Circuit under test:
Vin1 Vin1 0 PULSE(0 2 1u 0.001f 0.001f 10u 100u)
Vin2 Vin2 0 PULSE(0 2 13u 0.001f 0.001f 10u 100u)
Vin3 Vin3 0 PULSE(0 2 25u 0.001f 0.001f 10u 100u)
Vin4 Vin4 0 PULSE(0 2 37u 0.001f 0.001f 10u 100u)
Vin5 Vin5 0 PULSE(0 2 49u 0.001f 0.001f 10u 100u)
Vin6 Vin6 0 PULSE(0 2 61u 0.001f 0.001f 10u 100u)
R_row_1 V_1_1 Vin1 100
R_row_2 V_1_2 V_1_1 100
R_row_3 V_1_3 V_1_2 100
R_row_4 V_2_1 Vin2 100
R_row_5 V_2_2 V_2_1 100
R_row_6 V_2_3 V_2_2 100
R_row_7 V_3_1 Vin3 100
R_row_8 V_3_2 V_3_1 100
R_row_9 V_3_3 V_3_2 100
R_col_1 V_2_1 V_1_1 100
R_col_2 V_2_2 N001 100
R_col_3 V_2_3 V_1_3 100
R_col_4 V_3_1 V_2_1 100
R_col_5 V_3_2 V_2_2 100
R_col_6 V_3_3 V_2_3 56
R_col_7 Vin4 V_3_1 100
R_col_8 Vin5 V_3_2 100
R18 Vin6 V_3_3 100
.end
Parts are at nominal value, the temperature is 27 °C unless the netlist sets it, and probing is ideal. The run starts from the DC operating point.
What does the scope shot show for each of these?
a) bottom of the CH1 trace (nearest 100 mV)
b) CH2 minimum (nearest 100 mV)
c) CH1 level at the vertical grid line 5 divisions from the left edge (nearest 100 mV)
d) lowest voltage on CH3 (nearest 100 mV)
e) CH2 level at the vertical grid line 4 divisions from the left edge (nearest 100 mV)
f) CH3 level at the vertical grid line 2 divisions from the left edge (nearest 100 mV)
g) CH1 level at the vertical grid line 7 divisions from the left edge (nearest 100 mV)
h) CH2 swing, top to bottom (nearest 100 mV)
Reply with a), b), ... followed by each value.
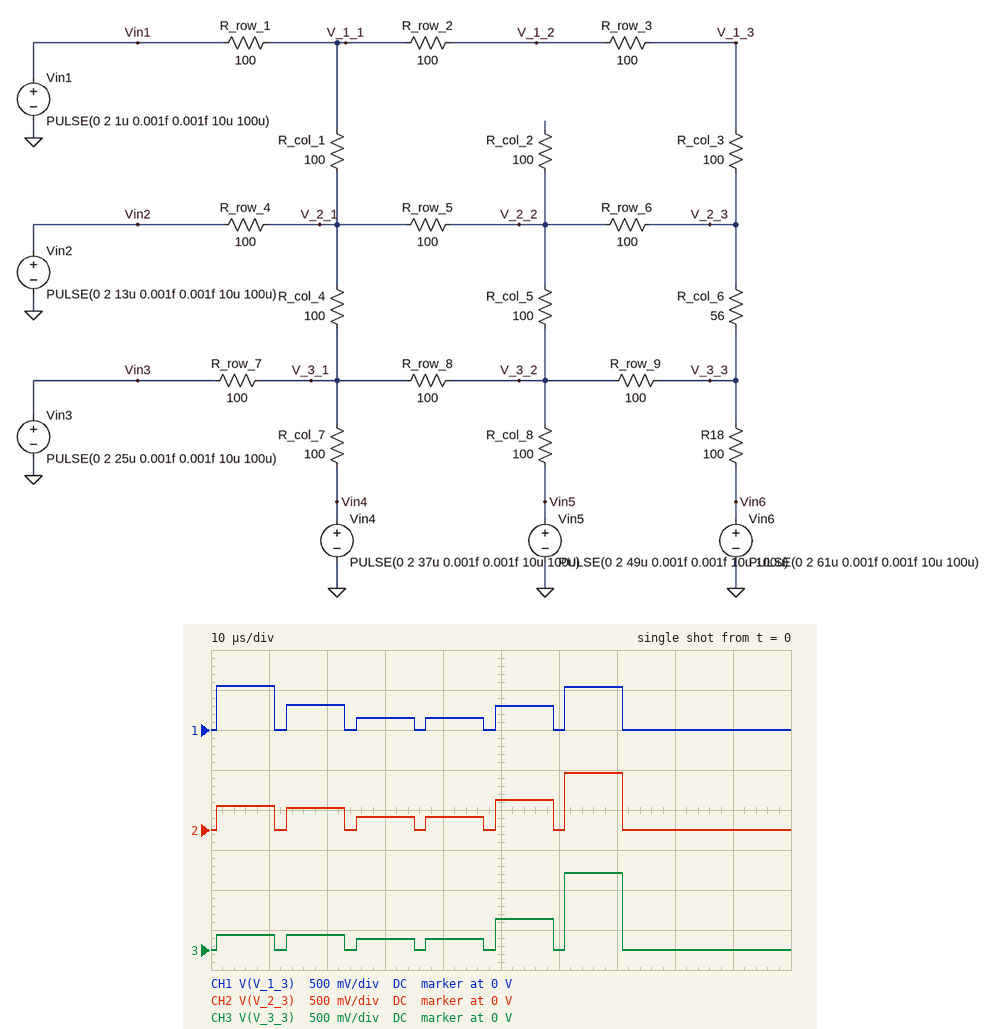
a) 0 V
b) 0 V
c) 300 mV
d) 0 V
e) 200 mV
f) 200 mV
g) 500 mV
h) 700 mV
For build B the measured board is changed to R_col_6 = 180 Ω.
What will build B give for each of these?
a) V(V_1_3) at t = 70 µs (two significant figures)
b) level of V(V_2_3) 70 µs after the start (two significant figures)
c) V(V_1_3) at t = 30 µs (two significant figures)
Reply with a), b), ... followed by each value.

a) 390 mV
b) 520 mV
c) 160 mV
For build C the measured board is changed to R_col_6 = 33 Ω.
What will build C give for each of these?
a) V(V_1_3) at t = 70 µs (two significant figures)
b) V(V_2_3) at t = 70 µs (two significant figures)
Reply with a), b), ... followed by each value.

a) 580 mV
b) 770 mV
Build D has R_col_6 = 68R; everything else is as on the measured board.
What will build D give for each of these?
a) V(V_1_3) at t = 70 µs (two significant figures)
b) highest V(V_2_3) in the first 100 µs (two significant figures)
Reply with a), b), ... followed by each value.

a) 510 mV
b) 680 mV
